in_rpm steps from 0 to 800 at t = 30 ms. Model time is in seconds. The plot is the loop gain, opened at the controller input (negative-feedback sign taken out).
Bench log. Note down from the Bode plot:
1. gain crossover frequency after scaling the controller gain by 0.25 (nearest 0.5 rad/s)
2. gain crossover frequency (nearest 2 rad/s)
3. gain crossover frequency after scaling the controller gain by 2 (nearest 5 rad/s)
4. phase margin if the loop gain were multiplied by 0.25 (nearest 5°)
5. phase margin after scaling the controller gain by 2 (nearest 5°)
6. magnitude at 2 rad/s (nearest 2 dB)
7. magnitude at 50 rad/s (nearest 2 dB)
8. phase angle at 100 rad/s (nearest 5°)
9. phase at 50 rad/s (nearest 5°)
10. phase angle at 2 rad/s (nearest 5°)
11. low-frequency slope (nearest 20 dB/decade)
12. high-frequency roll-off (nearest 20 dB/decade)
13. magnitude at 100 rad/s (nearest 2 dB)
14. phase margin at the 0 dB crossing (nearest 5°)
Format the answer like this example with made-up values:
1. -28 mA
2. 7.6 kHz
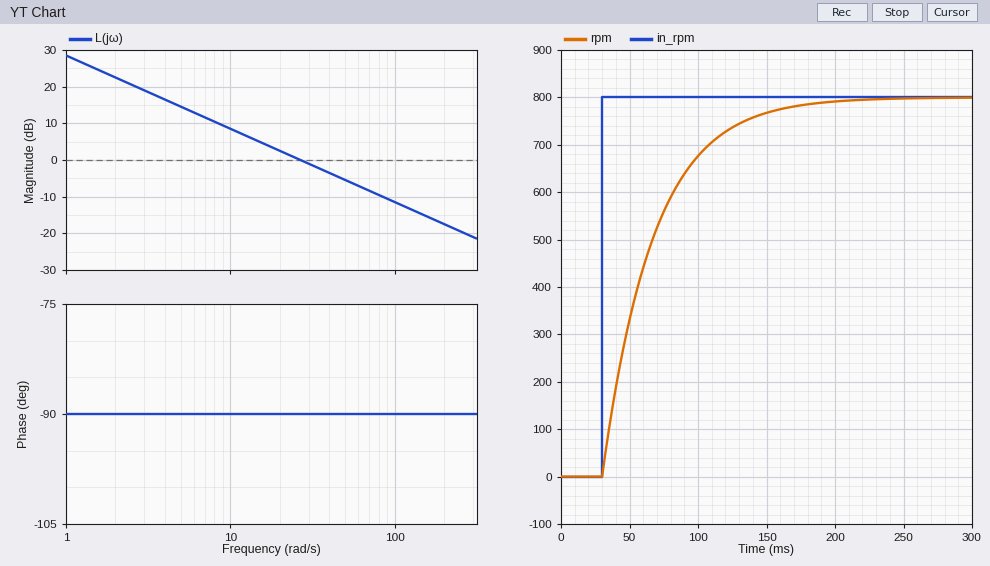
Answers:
1. 6.5 rad/s
2. 26 rad/s
3. 55 rad/s
4. 90°
5. 90°
6. 22 dB
7. -6 dB
8. -90°
9. -90°
10. -90°
11. -20 dB/decade
12. -20 dB/decade
13. -12 dB
14. 90°
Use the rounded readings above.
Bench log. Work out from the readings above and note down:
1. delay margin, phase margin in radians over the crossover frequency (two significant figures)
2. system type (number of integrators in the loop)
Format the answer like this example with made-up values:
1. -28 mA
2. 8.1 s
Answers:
1. 0.060 s
2. 1
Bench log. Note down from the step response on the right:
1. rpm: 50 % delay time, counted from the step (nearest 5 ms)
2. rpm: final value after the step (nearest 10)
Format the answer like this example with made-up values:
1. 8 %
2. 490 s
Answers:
1. 25 ms
2. 800
